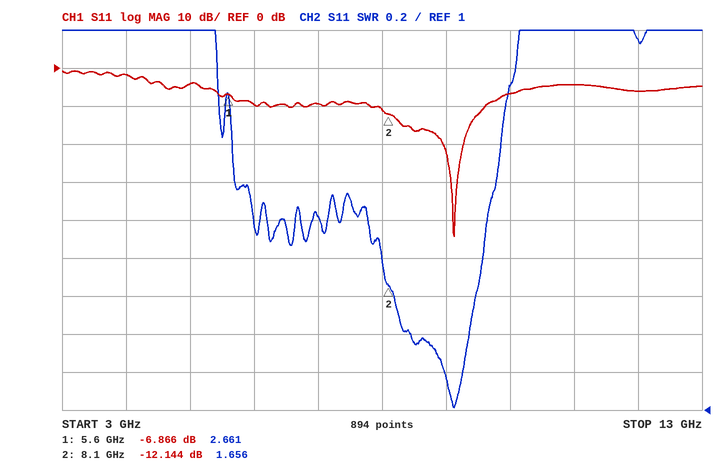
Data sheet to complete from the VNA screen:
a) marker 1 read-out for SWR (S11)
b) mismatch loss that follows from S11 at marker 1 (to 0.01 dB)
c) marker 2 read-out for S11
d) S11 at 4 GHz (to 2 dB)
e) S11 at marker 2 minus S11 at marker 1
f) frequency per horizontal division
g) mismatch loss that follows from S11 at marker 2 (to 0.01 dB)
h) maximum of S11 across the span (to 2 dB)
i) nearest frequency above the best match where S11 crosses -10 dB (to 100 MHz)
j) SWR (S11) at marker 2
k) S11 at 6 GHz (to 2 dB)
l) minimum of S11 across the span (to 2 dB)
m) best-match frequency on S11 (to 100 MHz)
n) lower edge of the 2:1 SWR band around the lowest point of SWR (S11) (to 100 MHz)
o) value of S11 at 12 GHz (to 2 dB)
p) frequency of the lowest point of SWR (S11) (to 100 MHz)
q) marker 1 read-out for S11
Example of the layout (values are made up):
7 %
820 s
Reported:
2.661
1.00 dB
-12.144 dB
-2 dB
-5.278 dB
1 GHz
0.27 dB
0 dB
9.6 GHz
1.656
-10 dB
-44 dB
9.1 GHz
7.8 GHz
-6 dB
9.1 GHz
-6.866 dB
